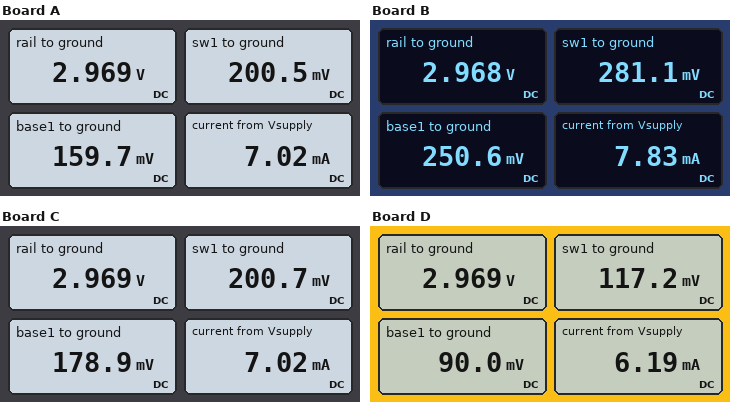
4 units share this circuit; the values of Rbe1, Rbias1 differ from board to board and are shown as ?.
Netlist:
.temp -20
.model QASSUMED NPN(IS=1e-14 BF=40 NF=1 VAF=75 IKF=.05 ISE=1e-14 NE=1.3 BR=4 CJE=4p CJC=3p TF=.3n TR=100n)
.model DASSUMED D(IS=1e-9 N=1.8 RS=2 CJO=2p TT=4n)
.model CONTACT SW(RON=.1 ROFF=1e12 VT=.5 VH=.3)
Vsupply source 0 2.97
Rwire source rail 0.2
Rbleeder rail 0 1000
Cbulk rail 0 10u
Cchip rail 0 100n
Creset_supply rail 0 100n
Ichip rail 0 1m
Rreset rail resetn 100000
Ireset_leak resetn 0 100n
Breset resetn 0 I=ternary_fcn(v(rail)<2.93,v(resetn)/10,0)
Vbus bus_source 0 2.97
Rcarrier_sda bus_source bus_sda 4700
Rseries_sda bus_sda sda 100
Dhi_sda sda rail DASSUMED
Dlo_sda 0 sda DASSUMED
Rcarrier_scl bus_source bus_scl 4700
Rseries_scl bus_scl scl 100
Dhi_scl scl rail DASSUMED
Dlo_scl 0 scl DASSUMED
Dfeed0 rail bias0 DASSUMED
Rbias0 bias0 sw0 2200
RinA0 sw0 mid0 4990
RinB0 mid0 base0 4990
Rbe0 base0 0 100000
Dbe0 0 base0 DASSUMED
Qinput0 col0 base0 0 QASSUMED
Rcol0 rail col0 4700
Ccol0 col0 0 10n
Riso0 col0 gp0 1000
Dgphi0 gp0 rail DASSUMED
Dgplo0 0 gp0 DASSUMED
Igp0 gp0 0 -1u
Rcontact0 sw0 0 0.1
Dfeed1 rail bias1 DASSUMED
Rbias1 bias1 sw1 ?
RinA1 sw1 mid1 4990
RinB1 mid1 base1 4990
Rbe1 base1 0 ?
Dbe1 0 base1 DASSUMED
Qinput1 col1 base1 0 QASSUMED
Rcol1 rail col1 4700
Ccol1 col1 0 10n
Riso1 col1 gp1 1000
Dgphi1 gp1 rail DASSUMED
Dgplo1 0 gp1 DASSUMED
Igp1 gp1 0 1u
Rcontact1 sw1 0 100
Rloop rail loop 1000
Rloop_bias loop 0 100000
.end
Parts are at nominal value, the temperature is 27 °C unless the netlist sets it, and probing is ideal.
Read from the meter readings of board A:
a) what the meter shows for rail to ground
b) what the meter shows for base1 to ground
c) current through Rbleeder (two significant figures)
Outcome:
2.969 V
159.7 mV
3.0 mA
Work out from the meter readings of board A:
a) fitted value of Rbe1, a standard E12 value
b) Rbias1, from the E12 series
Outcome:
39 kΩ
1 kΩ
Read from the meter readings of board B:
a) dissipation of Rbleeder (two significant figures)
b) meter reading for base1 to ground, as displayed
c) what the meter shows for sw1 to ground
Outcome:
8.8 mW
250.6 mV
281.1 mV
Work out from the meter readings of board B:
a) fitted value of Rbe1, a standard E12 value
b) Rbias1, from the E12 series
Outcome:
82 kΩ
680 Ω
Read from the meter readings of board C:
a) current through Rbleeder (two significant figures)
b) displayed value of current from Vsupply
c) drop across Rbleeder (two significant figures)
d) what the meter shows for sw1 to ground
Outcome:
3.0 mA
7.02 mA
3.0 V
200.7 mV
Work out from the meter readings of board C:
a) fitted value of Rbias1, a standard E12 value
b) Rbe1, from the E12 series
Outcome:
1 kΩ
82 kΩ
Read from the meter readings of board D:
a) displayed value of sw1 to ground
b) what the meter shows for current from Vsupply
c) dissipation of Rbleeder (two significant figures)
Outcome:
117.2 mV
6.19 mA
8.8 mW
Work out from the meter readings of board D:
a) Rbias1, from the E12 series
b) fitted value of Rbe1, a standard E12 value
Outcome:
1.8 kΩ
33 kΩ
